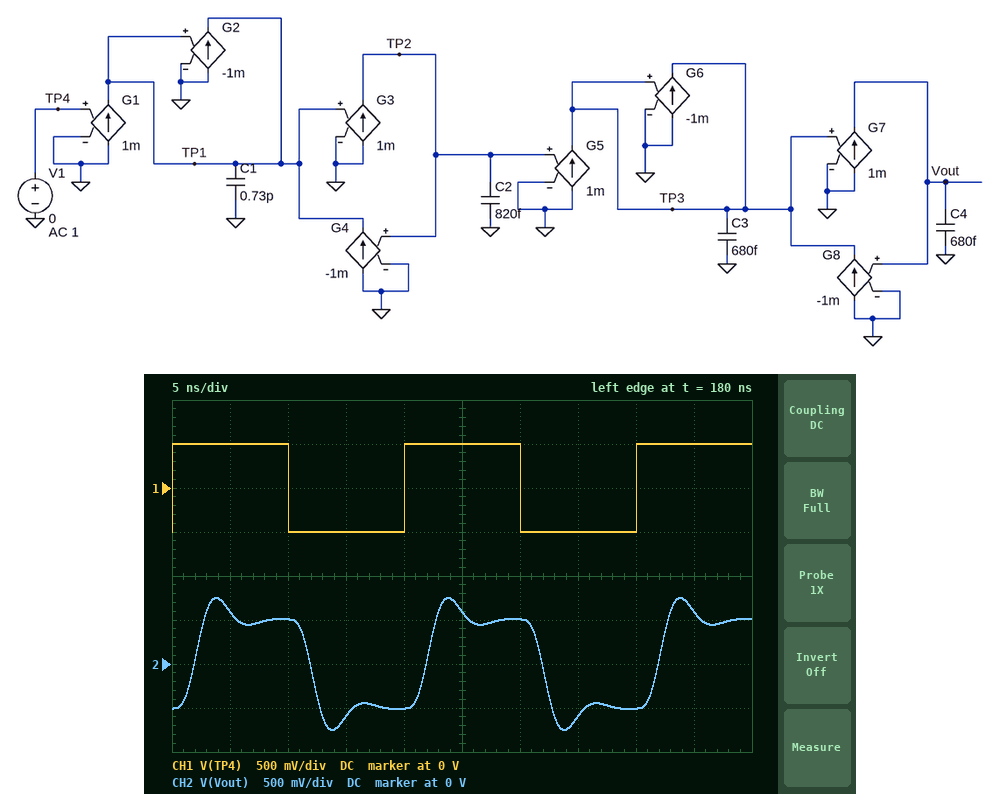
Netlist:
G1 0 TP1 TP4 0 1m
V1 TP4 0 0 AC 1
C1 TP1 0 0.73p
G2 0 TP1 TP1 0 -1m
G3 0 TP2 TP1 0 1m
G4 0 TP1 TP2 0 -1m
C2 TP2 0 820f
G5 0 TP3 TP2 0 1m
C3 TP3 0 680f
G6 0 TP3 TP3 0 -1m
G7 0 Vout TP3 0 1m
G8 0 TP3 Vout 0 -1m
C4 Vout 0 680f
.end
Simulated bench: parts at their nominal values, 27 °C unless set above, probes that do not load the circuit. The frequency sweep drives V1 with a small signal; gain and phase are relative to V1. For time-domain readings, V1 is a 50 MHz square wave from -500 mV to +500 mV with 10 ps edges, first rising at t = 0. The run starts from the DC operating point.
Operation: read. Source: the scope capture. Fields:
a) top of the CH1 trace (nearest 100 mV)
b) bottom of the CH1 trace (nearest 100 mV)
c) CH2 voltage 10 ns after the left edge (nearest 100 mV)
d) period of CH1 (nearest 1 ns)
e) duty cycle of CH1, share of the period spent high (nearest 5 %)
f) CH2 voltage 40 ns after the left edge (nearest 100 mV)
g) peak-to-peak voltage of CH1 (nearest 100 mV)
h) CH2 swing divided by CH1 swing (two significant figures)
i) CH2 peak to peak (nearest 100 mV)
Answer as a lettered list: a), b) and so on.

a) 500 mV
b) -500 mV
c) 500 mV
d) 20 ns
e) 50 %
f) -500 mV
g) 1.0 V
h) 1.5
i) 1.5 V
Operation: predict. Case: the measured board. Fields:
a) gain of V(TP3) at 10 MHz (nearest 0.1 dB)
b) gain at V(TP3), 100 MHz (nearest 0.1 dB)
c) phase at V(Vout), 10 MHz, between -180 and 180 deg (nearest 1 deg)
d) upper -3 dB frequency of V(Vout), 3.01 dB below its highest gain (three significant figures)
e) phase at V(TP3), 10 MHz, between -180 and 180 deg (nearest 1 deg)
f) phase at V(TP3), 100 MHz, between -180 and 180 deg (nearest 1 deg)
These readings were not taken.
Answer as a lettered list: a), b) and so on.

a) -27.4 dB
b) -6.0 dB
c) -5 deg
d) 223 MHz
e) 85 deg
f) 28 deg
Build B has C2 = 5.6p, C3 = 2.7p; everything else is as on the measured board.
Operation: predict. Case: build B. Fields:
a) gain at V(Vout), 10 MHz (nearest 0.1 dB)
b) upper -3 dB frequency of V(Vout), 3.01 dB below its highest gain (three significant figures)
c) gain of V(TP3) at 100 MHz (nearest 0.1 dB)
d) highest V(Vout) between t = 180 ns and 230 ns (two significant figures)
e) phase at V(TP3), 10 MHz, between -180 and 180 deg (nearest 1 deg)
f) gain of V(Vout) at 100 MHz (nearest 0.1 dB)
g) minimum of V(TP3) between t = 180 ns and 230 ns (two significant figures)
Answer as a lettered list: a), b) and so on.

a) -0.3 dB
b) 38.8 MHz
c) -12.6 dB
d) 360 mV
e) 68 deg
f) -5.2 dB
g) -110 mV
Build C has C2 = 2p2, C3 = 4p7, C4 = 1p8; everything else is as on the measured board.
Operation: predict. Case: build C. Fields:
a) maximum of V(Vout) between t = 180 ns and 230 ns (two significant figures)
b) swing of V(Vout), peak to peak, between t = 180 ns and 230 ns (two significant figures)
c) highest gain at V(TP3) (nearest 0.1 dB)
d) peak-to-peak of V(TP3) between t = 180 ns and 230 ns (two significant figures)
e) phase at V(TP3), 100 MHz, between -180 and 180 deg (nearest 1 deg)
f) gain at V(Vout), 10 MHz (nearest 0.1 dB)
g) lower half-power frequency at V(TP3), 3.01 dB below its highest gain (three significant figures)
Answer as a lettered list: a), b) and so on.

a) 990 mV
b) 2.0 V
c) -0.9 dB
d) 1.1 V
e) -139 deg
f) 0.2 dB
g) 39.2 MHz
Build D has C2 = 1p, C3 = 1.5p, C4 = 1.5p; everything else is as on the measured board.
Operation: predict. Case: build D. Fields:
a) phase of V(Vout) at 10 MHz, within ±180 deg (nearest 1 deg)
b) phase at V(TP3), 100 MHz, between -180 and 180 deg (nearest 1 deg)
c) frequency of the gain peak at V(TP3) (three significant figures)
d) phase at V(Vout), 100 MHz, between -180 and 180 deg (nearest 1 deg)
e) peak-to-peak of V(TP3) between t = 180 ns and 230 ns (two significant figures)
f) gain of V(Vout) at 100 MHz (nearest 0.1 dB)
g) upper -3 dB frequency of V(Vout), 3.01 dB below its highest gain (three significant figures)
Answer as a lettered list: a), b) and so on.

a) -9 deg
b) -35 deg
c) 106 MHz
d) -125 deg
e) 1.0 V
f) 0.9 dB
g) 124 MHz
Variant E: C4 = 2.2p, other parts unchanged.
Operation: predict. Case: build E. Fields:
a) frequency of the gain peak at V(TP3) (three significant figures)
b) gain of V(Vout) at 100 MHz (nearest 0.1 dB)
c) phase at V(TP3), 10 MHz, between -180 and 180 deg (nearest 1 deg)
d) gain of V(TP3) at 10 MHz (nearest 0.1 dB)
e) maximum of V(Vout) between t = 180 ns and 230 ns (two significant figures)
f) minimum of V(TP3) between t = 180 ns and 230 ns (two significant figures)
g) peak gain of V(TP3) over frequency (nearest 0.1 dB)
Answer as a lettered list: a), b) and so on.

a) 133 MHz
b) -2.5 dB
c) 79 deg
d) -17.2 dB
e) 500 mV
f) -710 mV
g) 0.9 dB
